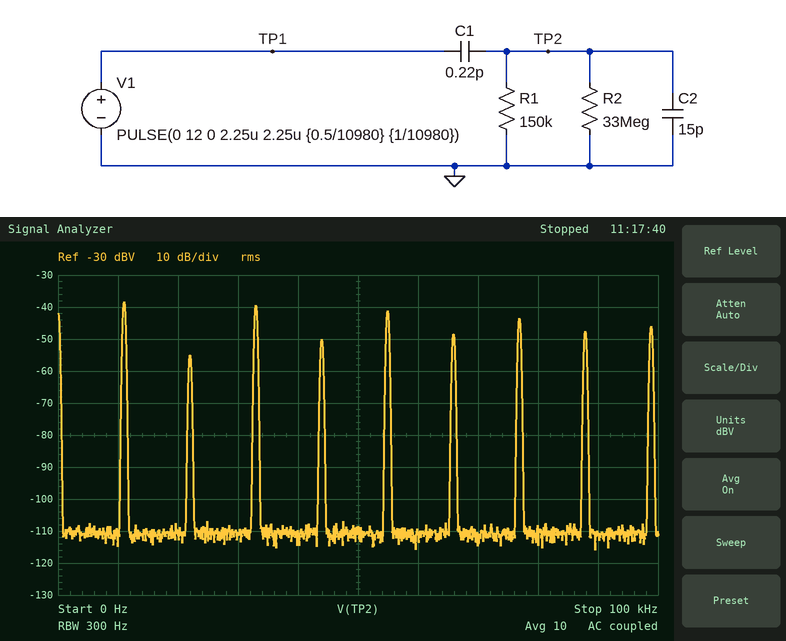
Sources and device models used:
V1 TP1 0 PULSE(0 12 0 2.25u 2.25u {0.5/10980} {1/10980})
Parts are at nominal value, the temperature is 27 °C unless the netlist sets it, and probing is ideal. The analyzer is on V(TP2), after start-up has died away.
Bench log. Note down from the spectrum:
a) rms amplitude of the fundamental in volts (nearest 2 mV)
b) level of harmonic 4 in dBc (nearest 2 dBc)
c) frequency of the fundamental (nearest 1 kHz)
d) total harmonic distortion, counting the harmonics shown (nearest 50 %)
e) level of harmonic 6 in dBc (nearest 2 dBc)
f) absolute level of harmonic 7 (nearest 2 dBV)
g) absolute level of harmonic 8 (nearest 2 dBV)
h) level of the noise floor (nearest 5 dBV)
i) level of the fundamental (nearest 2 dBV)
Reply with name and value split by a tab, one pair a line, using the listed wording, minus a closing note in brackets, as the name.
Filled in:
rms amplitude of the fundamental in volts	12 mV
level of harmonic 4 in dBc	-12 dBc
frequency of the fundamental	11 kHz
total harmonic distortion, counting the harmonics shown	150 %
level of harmonic 6 in dBc	-10 dBc
absolute level of harmonic 7	-44 dBV
absolute level of harmonic 8	-48 dBV
level of the noise floor	-110 dBV
level of the fundamental	-38 dBV
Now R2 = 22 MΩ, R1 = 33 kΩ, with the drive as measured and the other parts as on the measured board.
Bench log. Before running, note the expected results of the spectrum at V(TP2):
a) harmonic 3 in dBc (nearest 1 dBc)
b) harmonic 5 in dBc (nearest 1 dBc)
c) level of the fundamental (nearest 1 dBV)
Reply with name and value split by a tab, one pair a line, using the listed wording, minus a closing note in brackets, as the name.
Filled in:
harmonic 3 in dBc	0 dBc
harmonic 5 in dBc	-1 dBc
level of the fundamental	-51 dBV
